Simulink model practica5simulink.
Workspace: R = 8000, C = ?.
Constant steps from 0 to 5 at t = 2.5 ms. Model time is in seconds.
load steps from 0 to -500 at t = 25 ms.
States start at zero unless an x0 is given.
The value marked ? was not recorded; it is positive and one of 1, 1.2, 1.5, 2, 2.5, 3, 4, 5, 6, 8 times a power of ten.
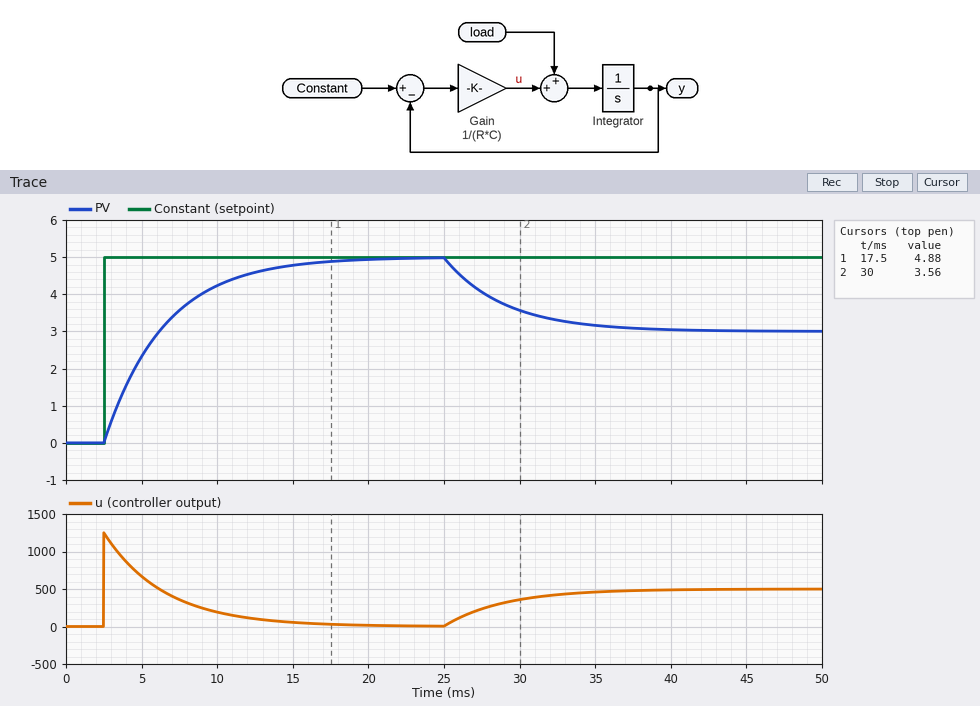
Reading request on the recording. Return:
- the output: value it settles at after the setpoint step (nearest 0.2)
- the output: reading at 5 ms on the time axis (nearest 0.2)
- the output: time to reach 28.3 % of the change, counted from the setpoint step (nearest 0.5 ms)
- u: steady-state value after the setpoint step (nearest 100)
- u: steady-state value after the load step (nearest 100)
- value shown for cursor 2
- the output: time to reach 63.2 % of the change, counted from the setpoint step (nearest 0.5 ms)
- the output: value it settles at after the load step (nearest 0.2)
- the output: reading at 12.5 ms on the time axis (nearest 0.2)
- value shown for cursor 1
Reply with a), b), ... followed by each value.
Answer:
a) 5.0
b) 2.4
c) 1.5 ms
d) 0
e) 500
f) 3.56
g) 4.0 ms
h) 3.0
i) 4.6
j) 4.88
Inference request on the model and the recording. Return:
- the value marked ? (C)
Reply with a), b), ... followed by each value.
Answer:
a) 5e-07
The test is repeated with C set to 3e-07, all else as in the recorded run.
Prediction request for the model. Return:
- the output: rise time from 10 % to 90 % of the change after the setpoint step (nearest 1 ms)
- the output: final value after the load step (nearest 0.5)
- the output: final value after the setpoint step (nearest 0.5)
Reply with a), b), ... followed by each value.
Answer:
a) 5 ms
b) 4.0
c) 5.0
